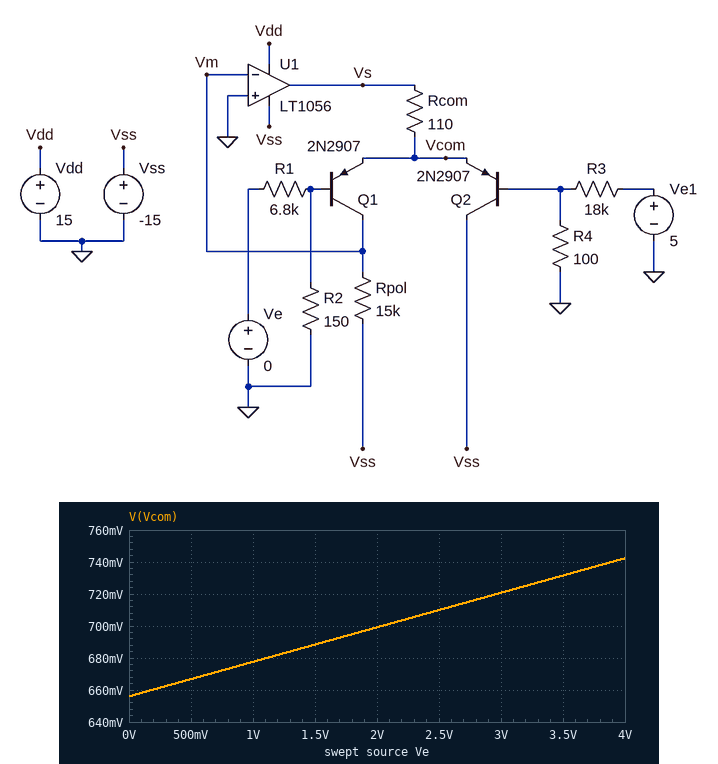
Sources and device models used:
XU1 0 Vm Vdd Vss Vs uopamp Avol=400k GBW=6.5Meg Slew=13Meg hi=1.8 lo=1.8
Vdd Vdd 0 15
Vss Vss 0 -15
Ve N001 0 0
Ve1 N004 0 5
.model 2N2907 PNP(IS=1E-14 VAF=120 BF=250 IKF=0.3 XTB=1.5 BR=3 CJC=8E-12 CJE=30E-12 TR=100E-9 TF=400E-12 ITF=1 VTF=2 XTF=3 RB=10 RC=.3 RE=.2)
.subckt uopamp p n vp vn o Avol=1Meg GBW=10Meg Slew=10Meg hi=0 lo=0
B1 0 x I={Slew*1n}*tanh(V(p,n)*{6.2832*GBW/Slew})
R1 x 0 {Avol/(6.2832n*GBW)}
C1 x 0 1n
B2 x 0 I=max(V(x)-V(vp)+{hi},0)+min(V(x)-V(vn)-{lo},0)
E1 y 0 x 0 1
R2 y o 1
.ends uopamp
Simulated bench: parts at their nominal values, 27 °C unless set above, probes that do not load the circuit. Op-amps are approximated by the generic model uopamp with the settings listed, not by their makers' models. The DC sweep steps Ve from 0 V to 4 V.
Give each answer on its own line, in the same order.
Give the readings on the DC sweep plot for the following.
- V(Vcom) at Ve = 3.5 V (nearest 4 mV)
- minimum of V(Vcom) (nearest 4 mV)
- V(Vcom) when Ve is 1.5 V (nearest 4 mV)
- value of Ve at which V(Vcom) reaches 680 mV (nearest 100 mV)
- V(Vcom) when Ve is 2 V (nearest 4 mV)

732 mV
656 mV
688 mV
1.1 V
700 mV
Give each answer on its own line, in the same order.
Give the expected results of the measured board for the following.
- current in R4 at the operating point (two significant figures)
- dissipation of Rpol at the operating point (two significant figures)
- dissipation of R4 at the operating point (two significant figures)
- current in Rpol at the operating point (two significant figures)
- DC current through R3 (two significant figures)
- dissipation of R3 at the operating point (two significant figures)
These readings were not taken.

280 µA
15 mW
7.7 µW
1.0 mA
280 µA
1.4 mW
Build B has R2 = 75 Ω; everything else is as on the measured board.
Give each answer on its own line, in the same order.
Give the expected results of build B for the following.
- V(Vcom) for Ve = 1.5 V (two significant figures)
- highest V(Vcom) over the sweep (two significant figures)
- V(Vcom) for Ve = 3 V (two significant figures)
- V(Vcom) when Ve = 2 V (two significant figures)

670 mV
700 mV
690 mV
680 mV
